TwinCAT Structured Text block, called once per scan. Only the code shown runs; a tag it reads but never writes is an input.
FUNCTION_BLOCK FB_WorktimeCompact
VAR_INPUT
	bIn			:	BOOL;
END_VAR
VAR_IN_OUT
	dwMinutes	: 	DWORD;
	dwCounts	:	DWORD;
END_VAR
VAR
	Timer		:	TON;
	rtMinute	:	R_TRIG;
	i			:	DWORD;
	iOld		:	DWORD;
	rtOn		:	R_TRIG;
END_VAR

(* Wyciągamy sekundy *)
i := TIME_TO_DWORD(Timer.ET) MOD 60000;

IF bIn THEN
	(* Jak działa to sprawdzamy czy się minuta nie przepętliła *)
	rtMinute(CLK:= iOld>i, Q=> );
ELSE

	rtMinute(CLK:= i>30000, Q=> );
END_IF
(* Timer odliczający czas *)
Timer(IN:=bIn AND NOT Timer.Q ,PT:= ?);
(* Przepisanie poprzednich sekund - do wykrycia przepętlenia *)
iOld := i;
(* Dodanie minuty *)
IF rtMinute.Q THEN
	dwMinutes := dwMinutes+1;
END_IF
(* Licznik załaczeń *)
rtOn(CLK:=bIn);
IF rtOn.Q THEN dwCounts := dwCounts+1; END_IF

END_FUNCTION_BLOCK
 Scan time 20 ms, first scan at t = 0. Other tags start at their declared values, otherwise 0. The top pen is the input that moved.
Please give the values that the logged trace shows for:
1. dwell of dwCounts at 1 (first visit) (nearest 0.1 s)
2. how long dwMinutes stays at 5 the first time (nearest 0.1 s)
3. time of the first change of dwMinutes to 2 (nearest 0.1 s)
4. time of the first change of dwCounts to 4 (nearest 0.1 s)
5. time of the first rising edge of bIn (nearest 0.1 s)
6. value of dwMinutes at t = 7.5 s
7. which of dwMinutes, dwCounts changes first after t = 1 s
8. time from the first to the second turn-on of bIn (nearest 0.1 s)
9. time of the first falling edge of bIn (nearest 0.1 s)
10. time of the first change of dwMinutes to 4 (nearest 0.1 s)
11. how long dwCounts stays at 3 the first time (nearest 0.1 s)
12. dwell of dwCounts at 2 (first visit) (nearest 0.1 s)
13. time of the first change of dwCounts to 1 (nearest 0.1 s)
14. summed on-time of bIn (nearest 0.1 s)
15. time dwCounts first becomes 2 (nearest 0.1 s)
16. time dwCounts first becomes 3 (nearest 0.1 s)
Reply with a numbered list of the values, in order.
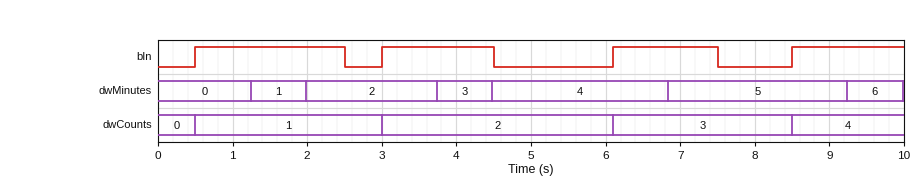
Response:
1. 2.5 s
2. 2.4 s
3. 2.0 s
4. 8.5 s
5. 0.5 s
6. 5
7. dwMinutes
8. 2.5 s
9. 2.5 s
10. 4.5 s
11. 2.4 s
12. 3.1 s
13. 0.5 s
14. 6.4 s
15. 3.0 s
16. 6.1 s
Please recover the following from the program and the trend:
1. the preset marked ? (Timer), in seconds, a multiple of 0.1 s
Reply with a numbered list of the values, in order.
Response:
1. 0.7 s
